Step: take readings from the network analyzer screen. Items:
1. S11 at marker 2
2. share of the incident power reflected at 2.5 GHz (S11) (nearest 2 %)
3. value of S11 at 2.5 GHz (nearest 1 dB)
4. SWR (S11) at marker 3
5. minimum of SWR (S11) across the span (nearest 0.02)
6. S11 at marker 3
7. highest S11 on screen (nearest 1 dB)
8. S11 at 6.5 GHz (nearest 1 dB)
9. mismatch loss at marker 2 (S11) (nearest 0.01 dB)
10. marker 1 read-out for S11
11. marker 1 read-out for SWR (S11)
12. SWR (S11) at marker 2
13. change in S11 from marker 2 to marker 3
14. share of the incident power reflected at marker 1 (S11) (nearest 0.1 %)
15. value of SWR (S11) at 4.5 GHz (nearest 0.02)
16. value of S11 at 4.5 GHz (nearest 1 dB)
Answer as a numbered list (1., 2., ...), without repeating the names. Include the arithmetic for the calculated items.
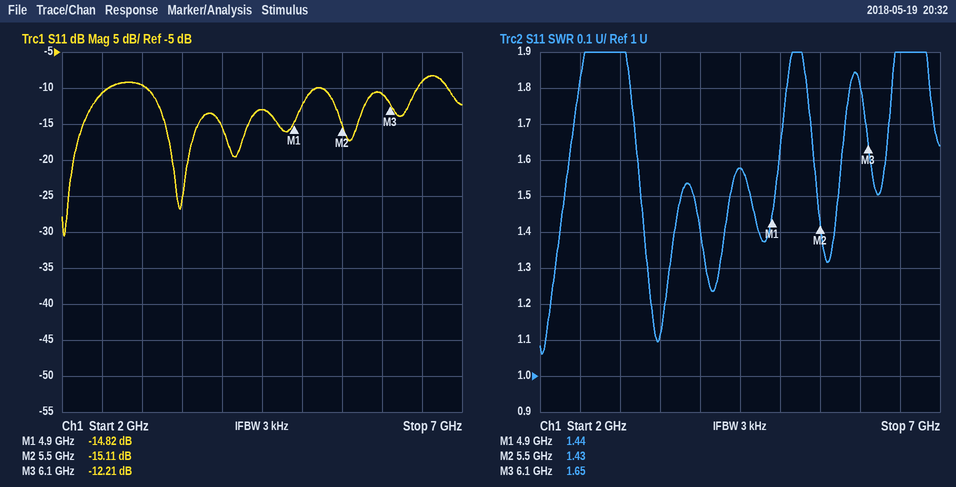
1. -15.11 dB
2. 10^(-11/10) ≈ 8 %
3. -11 dB
4. 1.65
5. 1.06
6. -12.21 dB
7. -8 dB
8. -9 dB
9. −10 log10(1 − 10^(-15.11/10)) ≈ 0.14 dB
10. -14.82 dB
11. 1.44
12. 1.43
13. -12.21 − (-15.11) = 2.90 dB
14. 10^(-14.82/10) ≈ 3.3 %
15. 1.58
16. -13 dB
